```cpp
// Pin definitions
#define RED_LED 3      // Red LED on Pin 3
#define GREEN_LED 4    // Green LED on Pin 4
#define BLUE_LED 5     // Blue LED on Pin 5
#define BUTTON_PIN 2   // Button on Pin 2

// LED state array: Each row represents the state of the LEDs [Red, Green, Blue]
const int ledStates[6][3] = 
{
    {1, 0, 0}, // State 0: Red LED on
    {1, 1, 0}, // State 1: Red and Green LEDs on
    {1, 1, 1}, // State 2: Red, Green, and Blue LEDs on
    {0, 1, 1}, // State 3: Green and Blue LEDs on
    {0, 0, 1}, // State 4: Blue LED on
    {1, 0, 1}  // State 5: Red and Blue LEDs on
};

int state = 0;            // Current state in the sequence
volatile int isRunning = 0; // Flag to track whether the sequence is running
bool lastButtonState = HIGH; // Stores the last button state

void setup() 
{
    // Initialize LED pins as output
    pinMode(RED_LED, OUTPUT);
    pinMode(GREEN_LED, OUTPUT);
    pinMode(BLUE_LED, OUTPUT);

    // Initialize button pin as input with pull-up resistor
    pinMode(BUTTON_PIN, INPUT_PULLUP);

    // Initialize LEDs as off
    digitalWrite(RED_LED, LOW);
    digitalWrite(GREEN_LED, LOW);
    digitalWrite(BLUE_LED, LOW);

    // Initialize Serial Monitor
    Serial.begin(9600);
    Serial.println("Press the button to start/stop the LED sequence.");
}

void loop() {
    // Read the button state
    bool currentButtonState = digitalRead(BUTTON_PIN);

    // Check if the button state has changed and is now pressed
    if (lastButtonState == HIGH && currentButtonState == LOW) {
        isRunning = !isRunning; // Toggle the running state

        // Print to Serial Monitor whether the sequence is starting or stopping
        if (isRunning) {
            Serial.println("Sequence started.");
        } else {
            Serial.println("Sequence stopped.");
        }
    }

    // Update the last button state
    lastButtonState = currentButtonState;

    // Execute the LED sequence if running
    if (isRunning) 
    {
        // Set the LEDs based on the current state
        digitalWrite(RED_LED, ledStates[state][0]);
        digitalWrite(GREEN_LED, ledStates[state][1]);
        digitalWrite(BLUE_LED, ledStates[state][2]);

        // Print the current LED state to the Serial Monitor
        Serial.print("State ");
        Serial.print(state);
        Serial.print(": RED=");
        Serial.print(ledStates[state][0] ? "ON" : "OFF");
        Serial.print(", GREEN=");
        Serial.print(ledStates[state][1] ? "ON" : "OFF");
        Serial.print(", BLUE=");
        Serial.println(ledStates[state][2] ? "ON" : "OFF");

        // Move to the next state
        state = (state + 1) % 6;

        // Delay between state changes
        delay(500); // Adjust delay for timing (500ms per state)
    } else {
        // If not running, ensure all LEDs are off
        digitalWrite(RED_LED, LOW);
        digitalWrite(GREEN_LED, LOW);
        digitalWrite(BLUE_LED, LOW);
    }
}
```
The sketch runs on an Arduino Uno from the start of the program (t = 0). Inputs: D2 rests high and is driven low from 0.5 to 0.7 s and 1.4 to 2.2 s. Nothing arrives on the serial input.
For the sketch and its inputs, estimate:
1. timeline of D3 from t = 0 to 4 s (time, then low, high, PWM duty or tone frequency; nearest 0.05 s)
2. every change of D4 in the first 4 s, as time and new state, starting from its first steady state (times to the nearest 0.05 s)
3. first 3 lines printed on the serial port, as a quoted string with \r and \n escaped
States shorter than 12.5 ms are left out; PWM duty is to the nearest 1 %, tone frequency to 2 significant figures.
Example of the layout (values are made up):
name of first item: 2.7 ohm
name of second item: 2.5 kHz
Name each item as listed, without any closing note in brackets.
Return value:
timeline of D3 from t = 0 to 4 s: 0 s low; 0.5 s high; 1.5 s low
every change of D4 in the first 4 s, as time and new state, starting from its first steady state: 0 s low; 1 s high; 1.5 s low
first 3 lines printed on the serial port, as a quoted string with \r and \n escaped: "Press the button to start/stop the LED sequence.\r\nSequence started.\r\nState 0: RED=ON, GREEN=OFF, BLUE=OFF\r\n"
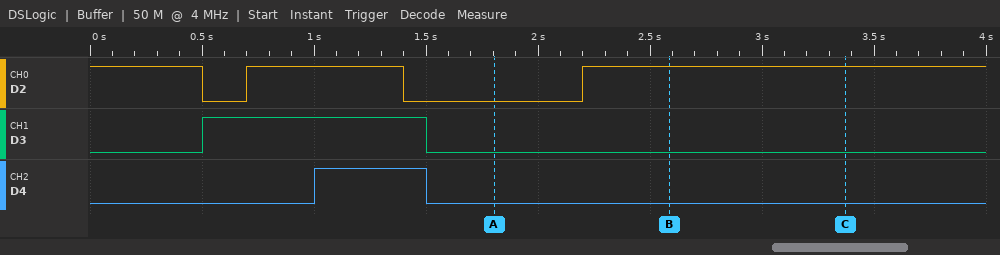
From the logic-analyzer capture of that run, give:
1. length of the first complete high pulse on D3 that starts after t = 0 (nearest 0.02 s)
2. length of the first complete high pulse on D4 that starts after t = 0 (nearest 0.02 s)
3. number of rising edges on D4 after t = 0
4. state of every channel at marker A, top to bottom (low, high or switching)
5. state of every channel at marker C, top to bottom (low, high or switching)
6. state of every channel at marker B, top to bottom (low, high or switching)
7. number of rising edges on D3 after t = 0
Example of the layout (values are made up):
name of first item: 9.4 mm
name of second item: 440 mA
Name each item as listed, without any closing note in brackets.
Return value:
length of the first complete high pulse on D3 that starts after t = 0: 1.00 s
length of the first complete high pulse on D4 that starts after t = 0: 0.50 s
number of rising edges on D4 after t = 0: 1
state of every channel at marker A, top to bottom: D2 low, D3 low, D4 low
state of every channel at marker C, top to bottom: D2 high, D3 low, D4 low
state of every channel at marker B, top to bottom: D2 high, D3 low, D4 low
number of rising edges on D3 after t = 0: 1
